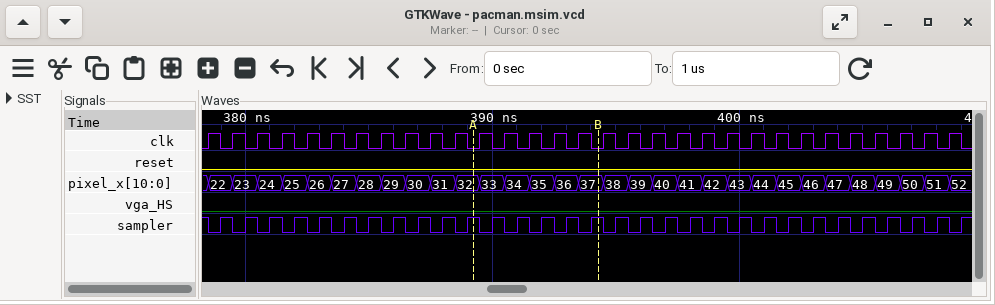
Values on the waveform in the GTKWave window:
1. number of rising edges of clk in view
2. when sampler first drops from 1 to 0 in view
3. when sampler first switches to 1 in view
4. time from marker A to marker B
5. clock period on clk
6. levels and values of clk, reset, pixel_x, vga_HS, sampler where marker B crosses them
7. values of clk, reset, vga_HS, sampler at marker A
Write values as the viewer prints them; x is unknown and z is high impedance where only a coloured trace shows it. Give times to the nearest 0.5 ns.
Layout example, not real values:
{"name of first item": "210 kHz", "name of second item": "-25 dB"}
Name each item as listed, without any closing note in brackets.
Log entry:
{"number of rising edges of clk in view": "31", "when sampler first drops from 1 to 0 in view": "378.5 ns", "when sampler first switches to 1 in view": "379 ns", "time from marker A to marker B": "5 ns", "clock period on clk": "1 ns", "levels and values of clk, reset, pixel_x, vga_HS, sampler where marker B crosses them": "clk=0, reset=0, pixel_x=37, vga_HS=0, sampler=1", "values of clk, reset, vga_HS, sampler at marker A": "clk=0, reset=0, vga_HS=0, sampler=1"}
